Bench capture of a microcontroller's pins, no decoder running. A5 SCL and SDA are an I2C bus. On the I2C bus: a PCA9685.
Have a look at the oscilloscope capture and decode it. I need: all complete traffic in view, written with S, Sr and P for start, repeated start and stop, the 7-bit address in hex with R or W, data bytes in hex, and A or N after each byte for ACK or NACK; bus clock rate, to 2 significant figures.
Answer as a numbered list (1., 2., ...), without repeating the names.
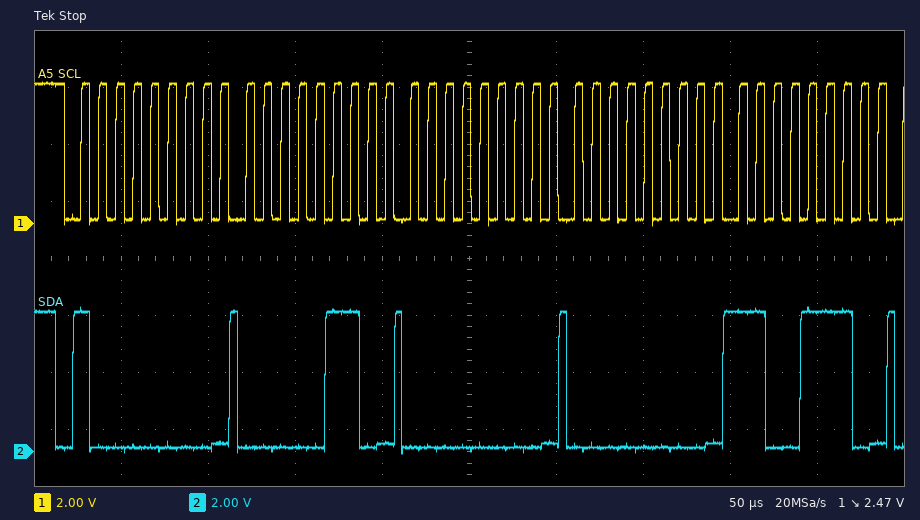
1. S 40W A 06 A 00 A 00 A CE A
2. 100 kHz
